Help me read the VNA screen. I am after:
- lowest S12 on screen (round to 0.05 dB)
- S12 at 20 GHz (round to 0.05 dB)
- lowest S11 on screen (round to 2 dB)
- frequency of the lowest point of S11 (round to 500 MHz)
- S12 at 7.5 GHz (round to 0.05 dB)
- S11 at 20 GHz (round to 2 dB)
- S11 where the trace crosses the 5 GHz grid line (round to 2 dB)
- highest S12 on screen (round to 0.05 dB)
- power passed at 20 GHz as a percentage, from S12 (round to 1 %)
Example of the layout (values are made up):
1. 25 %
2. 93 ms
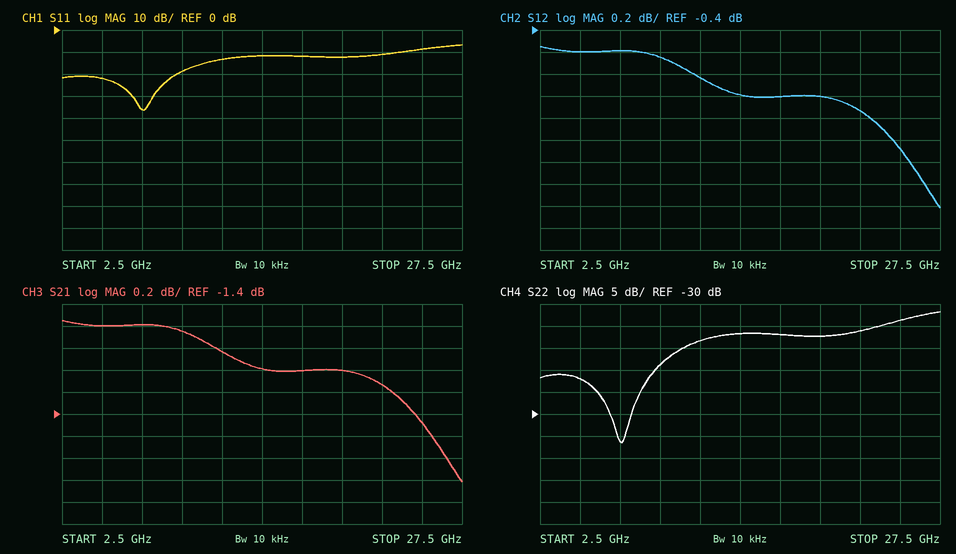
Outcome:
1. -2.00 dB
2. -1.00 dB
3. -36 dB
4. 7.5 GHz
5. -0.60 dB
6. -12 dB
7. -22 dB
8. -0.55 dB
9. 79 %
